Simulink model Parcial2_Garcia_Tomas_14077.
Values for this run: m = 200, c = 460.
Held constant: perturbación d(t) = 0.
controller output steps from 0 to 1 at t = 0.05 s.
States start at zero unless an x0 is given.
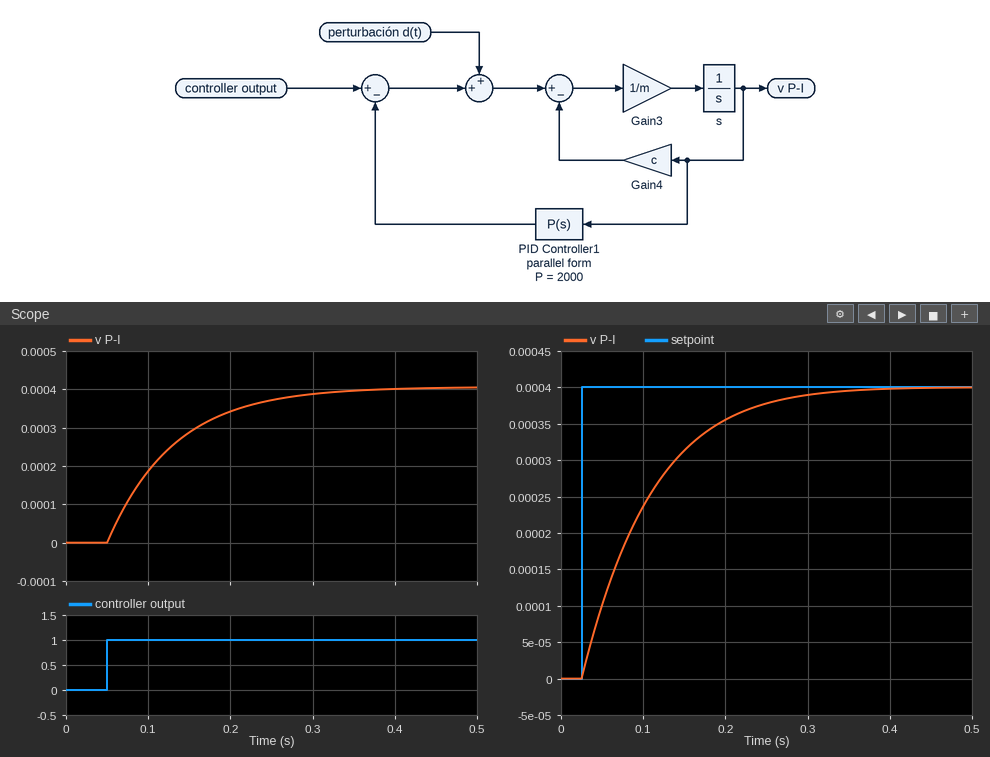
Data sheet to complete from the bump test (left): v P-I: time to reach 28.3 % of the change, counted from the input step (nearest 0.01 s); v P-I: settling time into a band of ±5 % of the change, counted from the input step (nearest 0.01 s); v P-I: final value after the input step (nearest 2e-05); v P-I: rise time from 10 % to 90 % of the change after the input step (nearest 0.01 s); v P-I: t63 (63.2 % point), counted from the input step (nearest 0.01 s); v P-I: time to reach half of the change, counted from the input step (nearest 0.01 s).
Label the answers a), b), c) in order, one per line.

a) 0.03 s
b) 0.24 s
c) 0.00040
d) 0.18 s
e) 0.08 s
f) 0.06 s
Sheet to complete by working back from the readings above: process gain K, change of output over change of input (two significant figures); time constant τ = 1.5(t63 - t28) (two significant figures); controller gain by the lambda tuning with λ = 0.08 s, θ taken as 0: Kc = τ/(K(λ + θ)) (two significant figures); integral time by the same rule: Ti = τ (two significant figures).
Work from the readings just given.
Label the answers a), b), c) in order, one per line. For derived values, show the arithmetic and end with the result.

a) (0.0004 - 0) / 1 = 0.00040
b) 1.5 × (0.08 - 0.03) = 0.075 s
c) 0.075 / (0.0004 × (0.08 + 0)) = 2300
d) 0.075 s
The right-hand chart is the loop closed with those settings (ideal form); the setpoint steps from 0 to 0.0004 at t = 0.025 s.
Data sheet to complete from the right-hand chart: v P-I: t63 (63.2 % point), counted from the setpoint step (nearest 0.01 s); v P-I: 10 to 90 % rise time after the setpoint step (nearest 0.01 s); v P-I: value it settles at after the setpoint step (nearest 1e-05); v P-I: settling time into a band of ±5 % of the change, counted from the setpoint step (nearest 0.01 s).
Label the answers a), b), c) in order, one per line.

a) 0.08 s
b) 0.17 s
c) 0.00040
d) 0.23 s
